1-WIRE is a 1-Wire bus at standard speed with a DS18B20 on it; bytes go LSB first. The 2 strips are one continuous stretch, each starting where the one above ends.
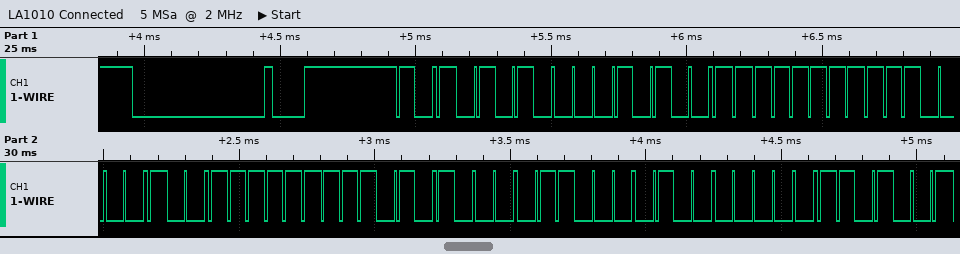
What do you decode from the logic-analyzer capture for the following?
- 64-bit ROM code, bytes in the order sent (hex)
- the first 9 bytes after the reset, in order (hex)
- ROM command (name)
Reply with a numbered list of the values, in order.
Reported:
1. 28 FF 87 FC 57 18 02 96
2. 55 28 FF 87 FC 57 18 02 96
3. Match ROM
